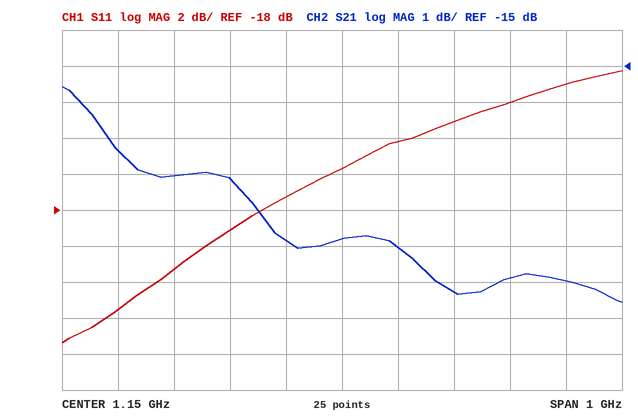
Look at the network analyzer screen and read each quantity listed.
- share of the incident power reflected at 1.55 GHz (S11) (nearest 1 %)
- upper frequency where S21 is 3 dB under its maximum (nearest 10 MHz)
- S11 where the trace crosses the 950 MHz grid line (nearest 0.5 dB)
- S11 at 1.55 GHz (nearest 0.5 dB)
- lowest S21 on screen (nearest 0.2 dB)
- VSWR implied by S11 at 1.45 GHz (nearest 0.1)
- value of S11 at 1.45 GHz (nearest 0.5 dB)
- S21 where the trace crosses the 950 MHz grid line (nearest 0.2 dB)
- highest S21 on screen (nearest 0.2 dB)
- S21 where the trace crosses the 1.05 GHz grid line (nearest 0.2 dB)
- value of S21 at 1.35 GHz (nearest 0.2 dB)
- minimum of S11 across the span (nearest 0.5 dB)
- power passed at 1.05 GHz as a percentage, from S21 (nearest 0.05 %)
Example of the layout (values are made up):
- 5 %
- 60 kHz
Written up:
- 8 %
- 980 MHz
- -19.0 dB
- -11.0 dB
- -21.6 dB
- 1.7
- -12.0 dB
- -18.2 dB
- -15.6 dB
- -19.8 dB
- -21.2 dB
- -25.5 dB
- 1.05 %
